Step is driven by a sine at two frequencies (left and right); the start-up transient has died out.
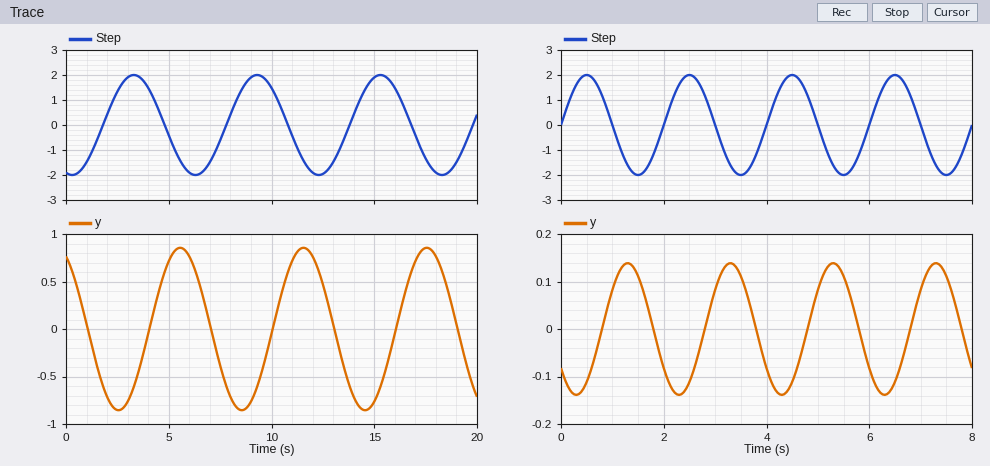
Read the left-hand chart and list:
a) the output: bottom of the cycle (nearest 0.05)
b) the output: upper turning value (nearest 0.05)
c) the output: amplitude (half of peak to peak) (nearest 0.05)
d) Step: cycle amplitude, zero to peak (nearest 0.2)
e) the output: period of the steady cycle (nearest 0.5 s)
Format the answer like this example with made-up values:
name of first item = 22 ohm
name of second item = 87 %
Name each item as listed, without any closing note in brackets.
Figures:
the output: bottom of the cycle = -0.85
the output: upper turning value = 0.85
the output: amplitude (half of peak to peak) = 0.85
Step: cycle amplitude, zero to peak = 2.0
the output: period of the steady cycle = 6.0 s
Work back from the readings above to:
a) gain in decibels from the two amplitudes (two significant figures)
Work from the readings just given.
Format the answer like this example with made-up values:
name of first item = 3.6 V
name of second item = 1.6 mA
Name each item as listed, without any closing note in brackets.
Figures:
gain in decibels from the two amplitudes = -7.4 dB
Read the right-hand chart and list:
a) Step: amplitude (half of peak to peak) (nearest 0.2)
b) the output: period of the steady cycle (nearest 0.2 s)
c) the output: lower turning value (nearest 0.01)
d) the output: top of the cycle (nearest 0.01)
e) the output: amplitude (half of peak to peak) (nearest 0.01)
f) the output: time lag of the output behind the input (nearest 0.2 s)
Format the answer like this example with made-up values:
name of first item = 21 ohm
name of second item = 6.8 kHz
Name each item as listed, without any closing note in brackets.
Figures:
Step: amplitude (half of peak to peak) = 2.0
the output: period of the steady cycle = 2.0 s
the output: lower turning value = -0.14
the output: top of the cycle = 0.14
the output: amplitude (half of peak to peak) = 0.14
the output: time lag of the output behind the input = 0.8 s
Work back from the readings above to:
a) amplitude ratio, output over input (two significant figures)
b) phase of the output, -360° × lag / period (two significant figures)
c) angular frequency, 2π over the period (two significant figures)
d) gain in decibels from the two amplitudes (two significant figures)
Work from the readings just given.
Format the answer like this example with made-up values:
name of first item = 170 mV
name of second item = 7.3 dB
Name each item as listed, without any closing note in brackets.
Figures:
amplitude ratio, output over input = 0.070
phase of the output, -360° × lag / period = -140°
angular frequency, 2π over the period = 3.1 rad/s
gain in decibels from the two amplitudes = -23 dB
